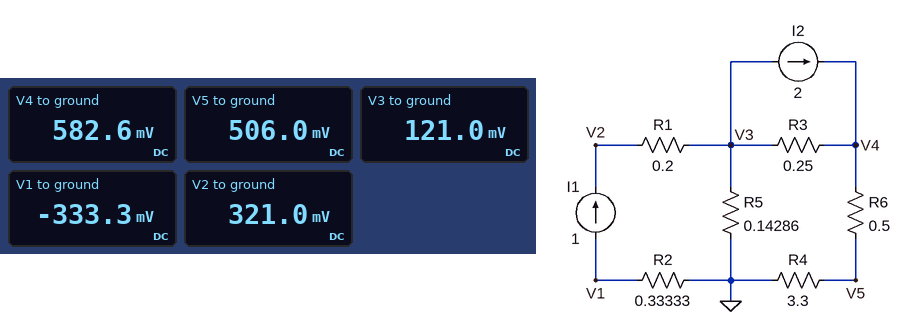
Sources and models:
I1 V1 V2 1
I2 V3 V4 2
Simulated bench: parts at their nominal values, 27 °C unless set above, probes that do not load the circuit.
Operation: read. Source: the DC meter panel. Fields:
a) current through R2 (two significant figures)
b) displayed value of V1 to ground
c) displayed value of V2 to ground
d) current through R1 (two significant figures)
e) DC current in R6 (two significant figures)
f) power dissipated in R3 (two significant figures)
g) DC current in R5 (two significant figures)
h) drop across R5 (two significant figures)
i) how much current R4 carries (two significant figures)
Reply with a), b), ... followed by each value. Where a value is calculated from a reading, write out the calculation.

a) (0 V - (-333.3 mV)) / 333.3 mΩ = 1.0 A
b) -333.3 mV
c) 321.0 mV
d) (321 mV - 121 mV) / 200 mΩ = 1.0 A
e) (582.6 mV - 506 mV) / 500 mΩ = 150 mA
f) (582.6 mV - 121 mV)^2 / 250 mΩ = 850 mW
g) (121 mV) / 142.9 mΩ = 850 mA
h) 121 mV = 120 mV
i) (506 mV) / 3.3 Ω = 150 mA
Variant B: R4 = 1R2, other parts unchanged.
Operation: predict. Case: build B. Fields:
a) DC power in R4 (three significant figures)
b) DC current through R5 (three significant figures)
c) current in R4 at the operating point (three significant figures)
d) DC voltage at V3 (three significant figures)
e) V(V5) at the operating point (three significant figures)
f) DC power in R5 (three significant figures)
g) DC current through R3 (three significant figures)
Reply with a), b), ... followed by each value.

a) 113 mW
b) 693 mA
c) 307 mA
d) 99.0 mV
e) 369 mV
f) 68.6 mW
g) 1.69 A
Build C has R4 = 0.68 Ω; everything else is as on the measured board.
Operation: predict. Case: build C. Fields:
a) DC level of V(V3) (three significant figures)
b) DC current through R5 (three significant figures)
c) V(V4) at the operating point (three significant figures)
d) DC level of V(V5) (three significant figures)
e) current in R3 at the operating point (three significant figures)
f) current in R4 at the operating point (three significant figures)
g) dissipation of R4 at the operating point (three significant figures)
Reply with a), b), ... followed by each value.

a) 84.5 mV
b) 591 mA
c) 482 mV
d) 278 mV
e) 1.59 A
f) 409 mA
g) 114 mW
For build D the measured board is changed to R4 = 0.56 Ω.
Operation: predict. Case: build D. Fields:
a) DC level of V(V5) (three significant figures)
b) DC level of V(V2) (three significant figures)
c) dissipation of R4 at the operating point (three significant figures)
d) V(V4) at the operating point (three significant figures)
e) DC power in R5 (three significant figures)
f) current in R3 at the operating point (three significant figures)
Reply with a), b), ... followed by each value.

a) 248 mV
b) 280 mV
c) 110 mW
d) 469 mV
e) 44.4 mW
f) 1.56 A
